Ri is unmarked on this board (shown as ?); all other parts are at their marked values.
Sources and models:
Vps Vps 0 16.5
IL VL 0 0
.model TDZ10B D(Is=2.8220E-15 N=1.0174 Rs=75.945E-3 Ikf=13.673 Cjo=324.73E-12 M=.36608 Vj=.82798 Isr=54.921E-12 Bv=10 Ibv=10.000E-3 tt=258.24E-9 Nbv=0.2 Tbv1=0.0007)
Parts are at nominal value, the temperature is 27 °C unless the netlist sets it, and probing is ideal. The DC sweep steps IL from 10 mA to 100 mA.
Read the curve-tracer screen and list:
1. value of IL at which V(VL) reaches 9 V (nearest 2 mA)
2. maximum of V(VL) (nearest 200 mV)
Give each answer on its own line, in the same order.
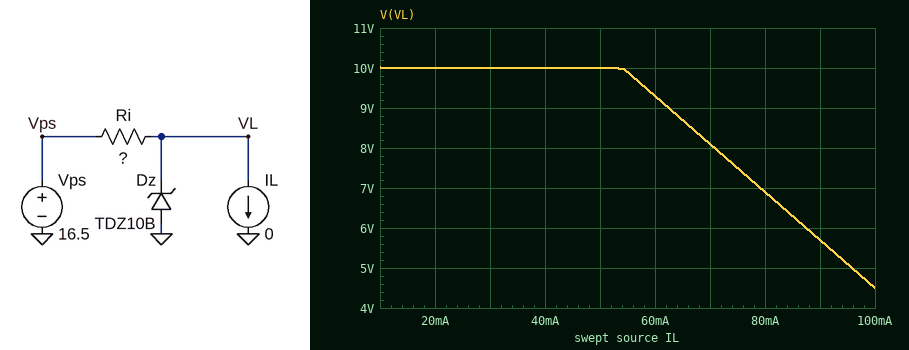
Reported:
62 mA
10.0 V
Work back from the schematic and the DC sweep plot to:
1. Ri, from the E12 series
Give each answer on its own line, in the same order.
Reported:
120 Ω
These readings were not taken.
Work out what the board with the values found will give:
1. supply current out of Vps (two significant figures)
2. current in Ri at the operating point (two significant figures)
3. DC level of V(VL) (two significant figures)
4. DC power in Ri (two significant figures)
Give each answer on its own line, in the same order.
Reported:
54 mA
54 mA
10 V
350 mW
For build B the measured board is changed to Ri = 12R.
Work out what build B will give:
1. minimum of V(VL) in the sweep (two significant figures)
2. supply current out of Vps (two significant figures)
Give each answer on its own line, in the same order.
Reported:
10 V
540 mA
